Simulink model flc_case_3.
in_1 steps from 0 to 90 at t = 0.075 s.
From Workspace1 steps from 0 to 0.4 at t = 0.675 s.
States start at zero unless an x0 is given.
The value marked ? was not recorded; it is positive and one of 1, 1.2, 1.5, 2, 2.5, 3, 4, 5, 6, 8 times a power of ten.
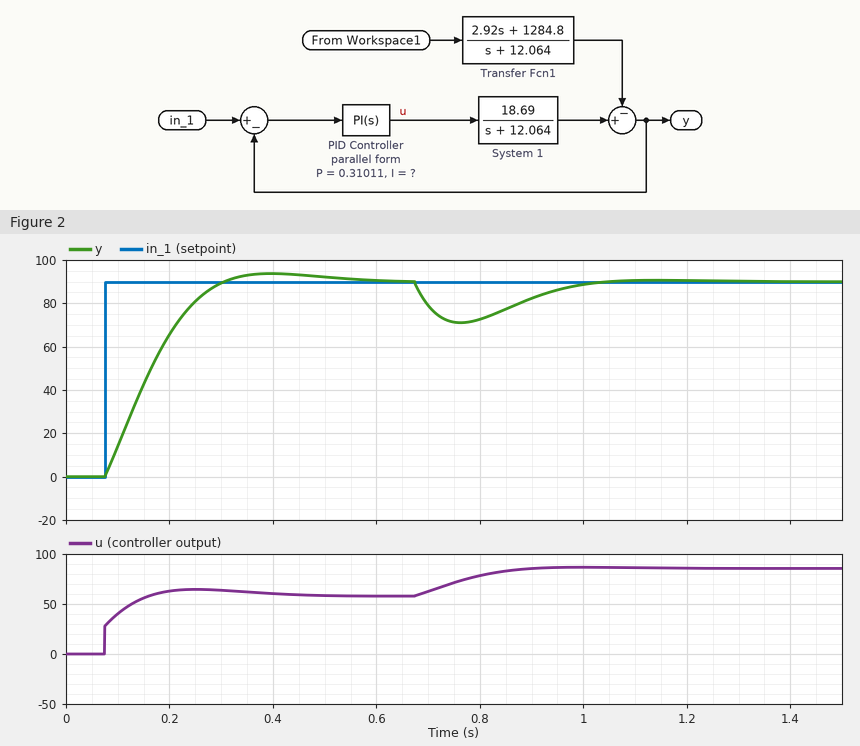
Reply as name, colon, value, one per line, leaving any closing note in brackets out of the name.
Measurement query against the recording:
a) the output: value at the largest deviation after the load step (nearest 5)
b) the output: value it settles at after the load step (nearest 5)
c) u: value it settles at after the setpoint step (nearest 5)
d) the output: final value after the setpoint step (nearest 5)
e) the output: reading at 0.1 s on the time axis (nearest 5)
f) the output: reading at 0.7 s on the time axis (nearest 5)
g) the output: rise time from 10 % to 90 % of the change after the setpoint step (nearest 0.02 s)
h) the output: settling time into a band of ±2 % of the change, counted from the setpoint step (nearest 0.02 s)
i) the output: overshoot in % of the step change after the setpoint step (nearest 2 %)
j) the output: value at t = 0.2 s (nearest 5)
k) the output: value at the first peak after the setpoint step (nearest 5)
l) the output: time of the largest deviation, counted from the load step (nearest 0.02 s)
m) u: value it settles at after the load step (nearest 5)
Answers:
the output: value at the largest deviation after the load step: 70
the output: value it settles at after the load step: 90
u: value it settles at after the setpoint step: 60
the output: final value after the setpoint step: 90
the output: reading at 0.1 s on the time axis: 15
the output: reading at 0.7 s on the time axis: 80
the output: rise time from 10 % to 90 % of the change after the setpoint step: 0.16 s
the output: settling time into a band of ±2 % of the change, counted from the setpoint step: 0.44 s
the output: overshoot in % of the step change after the setpoint step: 4 %
the output: value at t = 0.2 s: 65
the output: value at the first peak after the setpoint step: 95
the output: time of the largest deviation, counted from the load step: 0.08 s
u: value it settles at after the load step: 85
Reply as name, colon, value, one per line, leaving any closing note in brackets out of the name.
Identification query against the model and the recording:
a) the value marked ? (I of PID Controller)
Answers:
the value marked ?: 8
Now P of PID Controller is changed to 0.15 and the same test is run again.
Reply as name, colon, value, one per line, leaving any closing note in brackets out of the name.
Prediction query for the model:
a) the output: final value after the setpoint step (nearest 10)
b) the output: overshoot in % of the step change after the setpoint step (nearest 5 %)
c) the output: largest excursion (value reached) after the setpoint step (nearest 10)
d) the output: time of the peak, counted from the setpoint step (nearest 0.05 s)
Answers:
the output: final value after the setpoint step: 90
the output: overshoot in % of the step change after the setpoint step: 10 %
the output: largest excursion (value reached) after the setpoint step: 100
the output: time of the peak, counted from the setpoint step: 0.30 s
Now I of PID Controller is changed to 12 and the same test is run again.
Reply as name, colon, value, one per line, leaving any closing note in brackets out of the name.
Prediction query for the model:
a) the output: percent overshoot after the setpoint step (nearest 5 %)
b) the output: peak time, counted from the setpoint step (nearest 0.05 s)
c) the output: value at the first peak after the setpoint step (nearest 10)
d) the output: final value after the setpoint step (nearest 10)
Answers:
the output: percent overshoot after the setpoint step: 10 %
the output: peak time, counted from the setpoint step: 0.25 s
the output: value at the first peak after the setpoint step: 100
the output: final value after the setpoint step: 90
